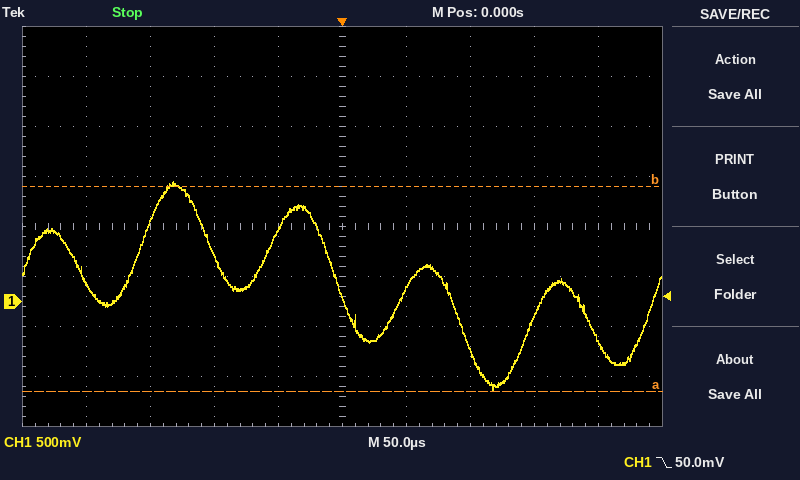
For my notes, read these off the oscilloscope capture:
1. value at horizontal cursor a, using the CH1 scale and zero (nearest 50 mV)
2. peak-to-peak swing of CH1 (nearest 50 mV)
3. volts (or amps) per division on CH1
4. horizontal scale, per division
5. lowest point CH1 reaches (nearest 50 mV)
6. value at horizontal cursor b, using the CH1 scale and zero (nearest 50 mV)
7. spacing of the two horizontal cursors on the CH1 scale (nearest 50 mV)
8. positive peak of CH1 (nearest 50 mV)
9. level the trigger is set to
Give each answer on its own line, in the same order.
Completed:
-900 mV
2.10 V
500 mV
50 µs
-900 mV
1.15 V
2.05 V
1.20 V
50.0 mV
